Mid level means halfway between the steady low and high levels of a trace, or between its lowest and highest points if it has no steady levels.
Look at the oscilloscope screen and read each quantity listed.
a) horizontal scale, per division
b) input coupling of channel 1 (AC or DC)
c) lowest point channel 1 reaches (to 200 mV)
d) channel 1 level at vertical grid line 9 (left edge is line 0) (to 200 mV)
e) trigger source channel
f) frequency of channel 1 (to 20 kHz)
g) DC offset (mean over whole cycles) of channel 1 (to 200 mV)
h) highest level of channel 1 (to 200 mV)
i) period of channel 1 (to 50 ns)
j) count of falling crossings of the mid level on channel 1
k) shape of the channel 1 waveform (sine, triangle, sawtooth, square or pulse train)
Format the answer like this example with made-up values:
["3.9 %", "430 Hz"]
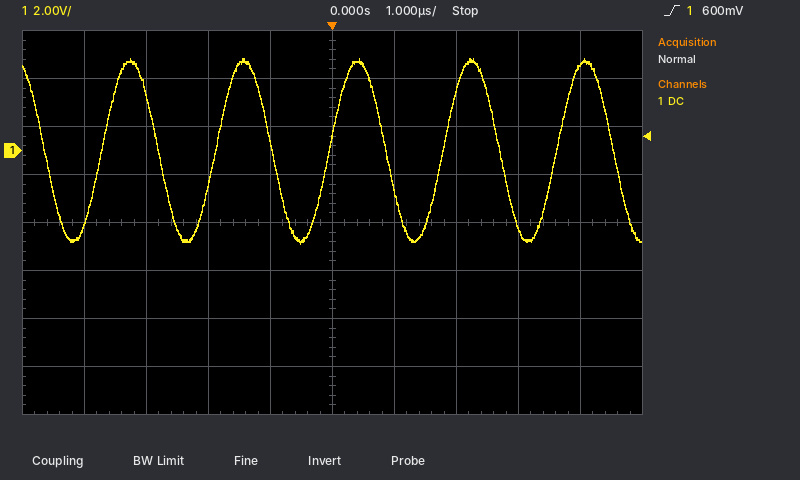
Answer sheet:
["1 µs", "DC", "-3.8 V", "3.6 V", "channel 1", "540 kHz", "0.0 V", "3.8 V", "1.85 µs", "6", "sine"]
